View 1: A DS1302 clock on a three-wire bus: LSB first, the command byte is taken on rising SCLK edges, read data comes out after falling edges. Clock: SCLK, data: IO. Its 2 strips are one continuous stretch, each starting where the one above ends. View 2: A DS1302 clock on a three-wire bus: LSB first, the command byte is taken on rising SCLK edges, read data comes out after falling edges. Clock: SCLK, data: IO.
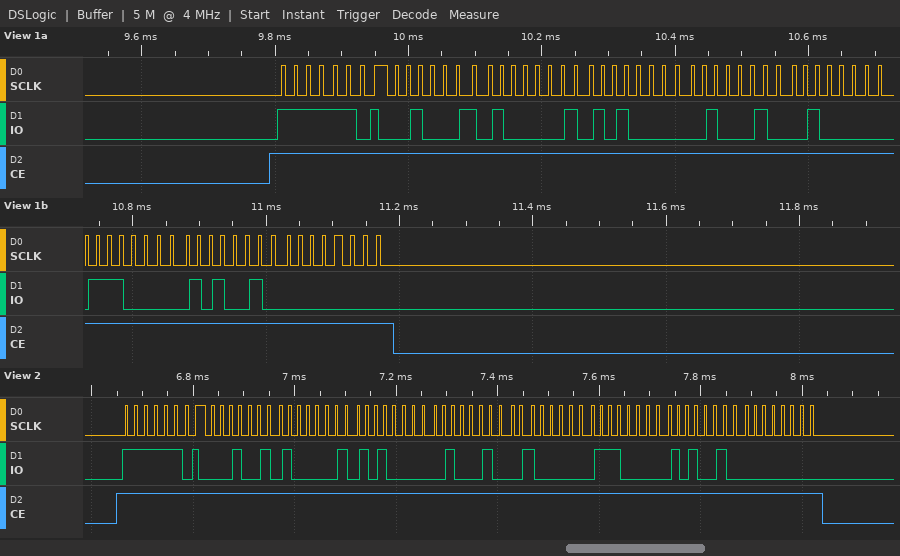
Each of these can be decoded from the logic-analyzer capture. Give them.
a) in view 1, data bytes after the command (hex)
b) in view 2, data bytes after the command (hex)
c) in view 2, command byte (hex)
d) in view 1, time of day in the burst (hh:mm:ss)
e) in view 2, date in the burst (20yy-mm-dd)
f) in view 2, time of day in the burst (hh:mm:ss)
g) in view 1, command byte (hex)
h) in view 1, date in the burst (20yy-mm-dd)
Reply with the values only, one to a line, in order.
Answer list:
44 41 05 22 02 07 25 00
48 41 05 22 02 07 25 00
0xBF
05:41:44
2025-02-22
05:41:48
0xBF
2025-02-22
